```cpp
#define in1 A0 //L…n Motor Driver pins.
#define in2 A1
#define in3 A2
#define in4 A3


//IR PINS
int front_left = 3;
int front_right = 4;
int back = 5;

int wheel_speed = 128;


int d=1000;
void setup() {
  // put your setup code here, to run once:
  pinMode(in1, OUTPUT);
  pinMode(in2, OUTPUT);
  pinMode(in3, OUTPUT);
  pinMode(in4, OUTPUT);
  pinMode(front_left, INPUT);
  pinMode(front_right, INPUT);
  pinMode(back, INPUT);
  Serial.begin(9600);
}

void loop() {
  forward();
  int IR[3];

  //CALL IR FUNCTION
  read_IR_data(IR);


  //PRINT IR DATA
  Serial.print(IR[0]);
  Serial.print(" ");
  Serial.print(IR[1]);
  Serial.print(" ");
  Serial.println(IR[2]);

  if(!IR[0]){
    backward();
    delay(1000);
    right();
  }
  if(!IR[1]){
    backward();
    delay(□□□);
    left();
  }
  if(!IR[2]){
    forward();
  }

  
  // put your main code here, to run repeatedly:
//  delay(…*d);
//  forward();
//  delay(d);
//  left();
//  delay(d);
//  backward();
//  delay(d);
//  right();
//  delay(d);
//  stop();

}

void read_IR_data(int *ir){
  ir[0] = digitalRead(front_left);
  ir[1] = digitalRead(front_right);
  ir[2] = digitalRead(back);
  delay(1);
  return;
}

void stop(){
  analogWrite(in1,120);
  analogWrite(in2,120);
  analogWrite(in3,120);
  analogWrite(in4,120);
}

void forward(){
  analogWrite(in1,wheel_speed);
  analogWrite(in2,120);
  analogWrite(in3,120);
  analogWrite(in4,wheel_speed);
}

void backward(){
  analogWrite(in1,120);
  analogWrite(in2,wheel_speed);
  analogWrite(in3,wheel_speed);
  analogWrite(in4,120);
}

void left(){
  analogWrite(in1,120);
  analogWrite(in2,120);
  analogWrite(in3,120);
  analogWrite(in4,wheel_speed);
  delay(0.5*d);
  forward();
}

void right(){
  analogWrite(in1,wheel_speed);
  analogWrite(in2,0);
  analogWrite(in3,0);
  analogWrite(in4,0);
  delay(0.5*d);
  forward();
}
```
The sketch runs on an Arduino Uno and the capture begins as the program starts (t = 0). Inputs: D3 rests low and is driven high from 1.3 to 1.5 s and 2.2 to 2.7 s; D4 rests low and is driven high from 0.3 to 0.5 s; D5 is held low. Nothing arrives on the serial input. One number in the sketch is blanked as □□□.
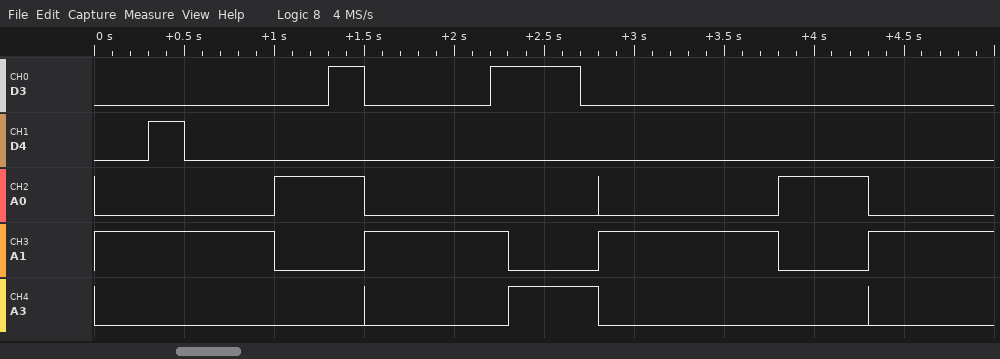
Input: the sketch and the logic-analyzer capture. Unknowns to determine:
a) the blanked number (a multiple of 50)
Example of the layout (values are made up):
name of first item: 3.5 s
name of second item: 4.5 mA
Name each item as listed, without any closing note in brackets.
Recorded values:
the blanked number: 800
